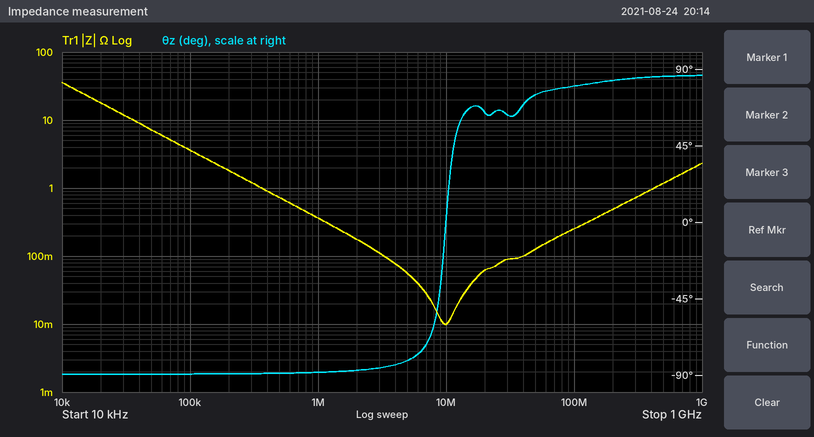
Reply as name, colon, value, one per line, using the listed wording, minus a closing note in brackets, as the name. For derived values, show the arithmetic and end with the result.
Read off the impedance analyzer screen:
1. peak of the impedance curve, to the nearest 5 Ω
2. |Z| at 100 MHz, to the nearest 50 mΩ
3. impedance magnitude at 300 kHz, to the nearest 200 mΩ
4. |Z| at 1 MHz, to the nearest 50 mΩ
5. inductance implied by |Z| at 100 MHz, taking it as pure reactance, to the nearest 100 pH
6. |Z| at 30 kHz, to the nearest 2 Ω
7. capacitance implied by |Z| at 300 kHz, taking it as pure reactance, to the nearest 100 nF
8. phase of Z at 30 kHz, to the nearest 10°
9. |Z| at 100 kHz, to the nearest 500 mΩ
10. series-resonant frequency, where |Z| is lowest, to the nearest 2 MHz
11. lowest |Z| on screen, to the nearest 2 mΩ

peak of the impedance curve, to the nearest 5 Ω: 35 Ω
|Z| at 100 MHz, to the nearest 50 mΩ: 250 mΩ
impedance magnitude at 300 kHz, to the nearest 200 mΩ: 1.2 Ω
|Z| at 1 MHz, to the nearest 50 mΩ: 350 mΩ
inductance implied by |Z| at 100 MHz, taking it as pure reactance, to the nearest 100 pH: L = 250 mΩ/(2π × 100 MHz) ≈ 398 pH, so 400 pH to the nearest 100 pH
|Z| at 30 kHz, to the nearest 2 Ω: 12 Ω
capacitance implied by |Z| at 300 kHz, taking it as pure reactance, to the nearest 100 nF: C = 1/(2π × 300 kHz × 1.2 Ω) ≈ 442 nF, so 400 nF to the nearest 100 nF
phase of Z at 30 kHz, to the nearest 10°: -90°
|Z| at 100 kHz, to the nearest 500 mΩ: 3.5 Ω
series-resonant frequency, where |Z| is lowest, to the nearest 2 MHz: 10 MHz
lowest |Z| on screen, to the nearest 2 mΩ: 10 mΩ
